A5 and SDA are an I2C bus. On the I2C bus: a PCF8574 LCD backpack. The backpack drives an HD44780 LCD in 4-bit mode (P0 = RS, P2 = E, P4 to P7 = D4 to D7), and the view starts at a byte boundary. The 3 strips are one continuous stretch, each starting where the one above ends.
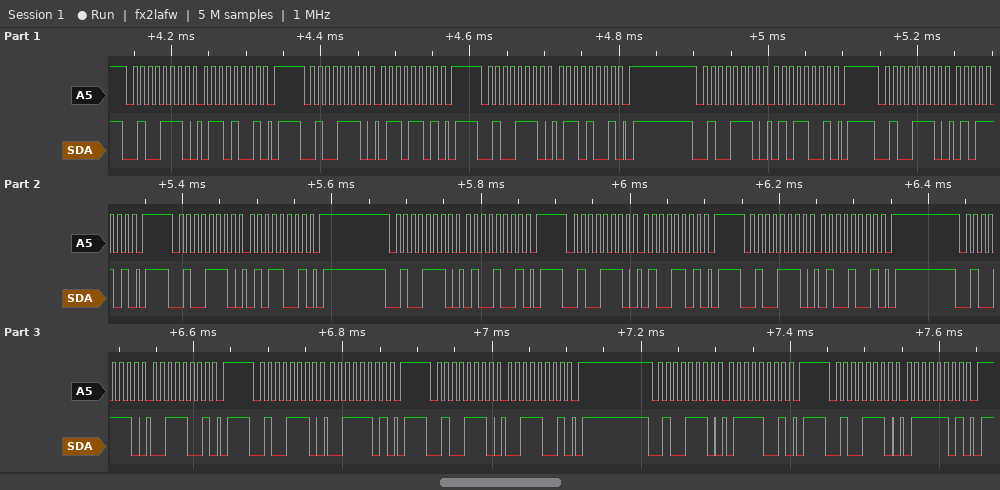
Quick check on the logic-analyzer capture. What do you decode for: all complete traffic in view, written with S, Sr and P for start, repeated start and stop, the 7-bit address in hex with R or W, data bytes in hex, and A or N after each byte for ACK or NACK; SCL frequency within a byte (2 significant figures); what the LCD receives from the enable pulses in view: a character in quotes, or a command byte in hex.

S 27W A 69 A P S 27W A 6D A P S 27W A 69 A P S 27W A 59 A P S 27W A 5D A P S 27W A 59 A P S 27W A 49 A P S 27W A 4D A P S 27W A 49 A P S 27W A 39 A P S 27W A 3D A P S 27W A 39 A P S 27W A 79 A P S 27W A 7D A P
100 kHz
'e' 'C'
